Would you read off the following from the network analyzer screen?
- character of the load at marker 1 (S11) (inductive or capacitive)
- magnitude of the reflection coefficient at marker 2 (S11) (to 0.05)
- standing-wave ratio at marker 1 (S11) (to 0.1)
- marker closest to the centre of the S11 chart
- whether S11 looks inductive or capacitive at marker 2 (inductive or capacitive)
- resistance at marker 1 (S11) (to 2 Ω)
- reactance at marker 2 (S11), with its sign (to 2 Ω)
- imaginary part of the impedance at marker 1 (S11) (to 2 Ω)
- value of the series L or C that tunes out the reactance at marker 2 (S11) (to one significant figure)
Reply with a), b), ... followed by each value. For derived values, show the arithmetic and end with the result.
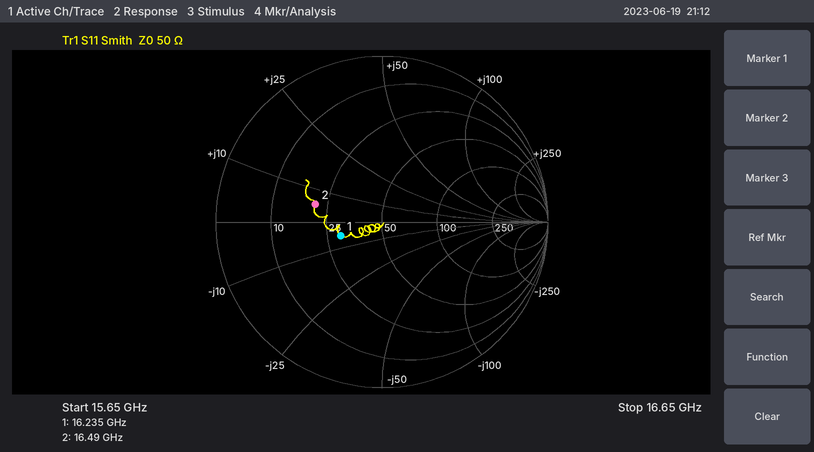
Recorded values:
a) capacitive
b) 0.40
c) 1.7
d) marker 1
e) inductive
f) 30 Ω
g) +6 Ω
h) -6 Ω
i) C = 1/(2π × 16.49 GHz × 6 Ω) ≈ 2 pF
